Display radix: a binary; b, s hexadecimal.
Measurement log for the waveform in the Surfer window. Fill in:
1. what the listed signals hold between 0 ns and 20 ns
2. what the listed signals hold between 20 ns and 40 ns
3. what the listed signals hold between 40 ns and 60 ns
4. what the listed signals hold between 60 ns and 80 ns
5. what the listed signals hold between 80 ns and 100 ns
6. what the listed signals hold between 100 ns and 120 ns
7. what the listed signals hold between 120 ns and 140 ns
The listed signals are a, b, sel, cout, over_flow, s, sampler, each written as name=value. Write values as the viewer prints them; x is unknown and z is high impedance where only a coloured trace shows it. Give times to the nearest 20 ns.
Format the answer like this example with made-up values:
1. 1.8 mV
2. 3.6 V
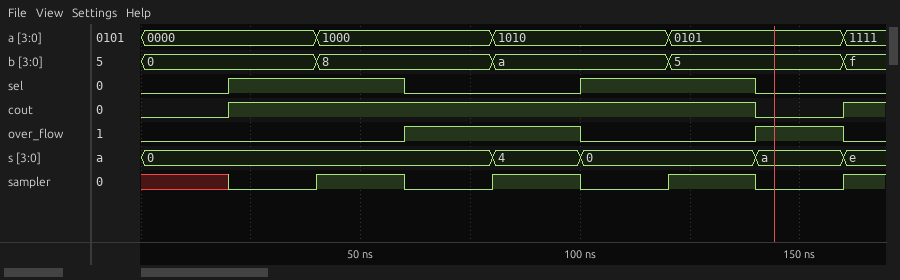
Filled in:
1. a=0000, b=0, sel=0, cout=0, over_flow=0, s=0, sampler=x
2. a=0000, b=0, sel=1, cout=1, over_flow=0, s=0, sampler=0
3. a=1000, b=8, sel=1, cout=1, over_flow=0, s=0, sampler=1
4. a=1000, b=8, sel=0, cout=1, over_flow=1, s=0, sampler=0
5. a=1010, b=a, sel=0, cout=1, over_flow=1, s=4, sampler=1
6. a=1010, b=a, sel=1, cout=1, over_flow=0, s=0, sampler=0
7. a=0101, b=5, sel=1, cout=1, over_flow=0, s=0, sampler=1
